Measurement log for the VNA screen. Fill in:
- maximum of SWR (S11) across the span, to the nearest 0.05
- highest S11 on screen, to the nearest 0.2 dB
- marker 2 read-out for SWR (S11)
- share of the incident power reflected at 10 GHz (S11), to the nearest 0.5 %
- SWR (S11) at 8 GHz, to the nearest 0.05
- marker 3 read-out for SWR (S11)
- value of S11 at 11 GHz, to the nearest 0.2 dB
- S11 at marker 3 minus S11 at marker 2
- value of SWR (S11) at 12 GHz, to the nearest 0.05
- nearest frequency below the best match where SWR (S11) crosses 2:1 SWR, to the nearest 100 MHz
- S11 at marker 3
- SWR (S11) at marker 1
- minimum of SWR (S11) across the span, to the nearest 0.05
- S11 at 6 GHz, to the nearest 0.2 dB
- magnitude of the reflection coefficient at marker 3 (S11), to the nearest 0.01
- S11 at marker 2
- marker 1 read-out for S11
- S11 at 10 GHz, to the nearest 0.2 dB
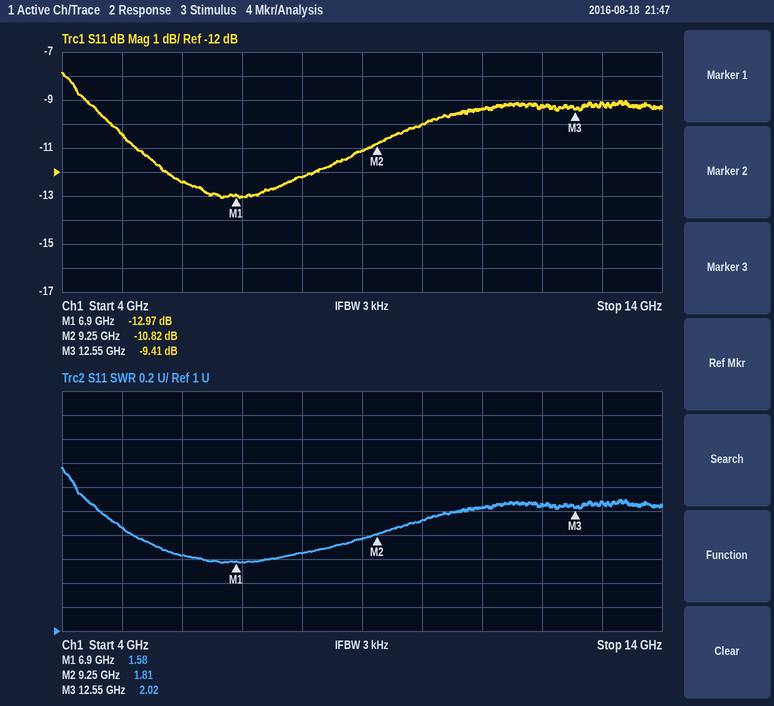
2.35
-7.8 dB
1.81
10.0 %
1.65
2.02
-9.4 dB
1.41 dB
2.05
4.6 GHz
-9.41 dB
1.58
1.55
-12.4 dB
0.34
-10.82 dB
-12.97 dB
-10.0 dB
